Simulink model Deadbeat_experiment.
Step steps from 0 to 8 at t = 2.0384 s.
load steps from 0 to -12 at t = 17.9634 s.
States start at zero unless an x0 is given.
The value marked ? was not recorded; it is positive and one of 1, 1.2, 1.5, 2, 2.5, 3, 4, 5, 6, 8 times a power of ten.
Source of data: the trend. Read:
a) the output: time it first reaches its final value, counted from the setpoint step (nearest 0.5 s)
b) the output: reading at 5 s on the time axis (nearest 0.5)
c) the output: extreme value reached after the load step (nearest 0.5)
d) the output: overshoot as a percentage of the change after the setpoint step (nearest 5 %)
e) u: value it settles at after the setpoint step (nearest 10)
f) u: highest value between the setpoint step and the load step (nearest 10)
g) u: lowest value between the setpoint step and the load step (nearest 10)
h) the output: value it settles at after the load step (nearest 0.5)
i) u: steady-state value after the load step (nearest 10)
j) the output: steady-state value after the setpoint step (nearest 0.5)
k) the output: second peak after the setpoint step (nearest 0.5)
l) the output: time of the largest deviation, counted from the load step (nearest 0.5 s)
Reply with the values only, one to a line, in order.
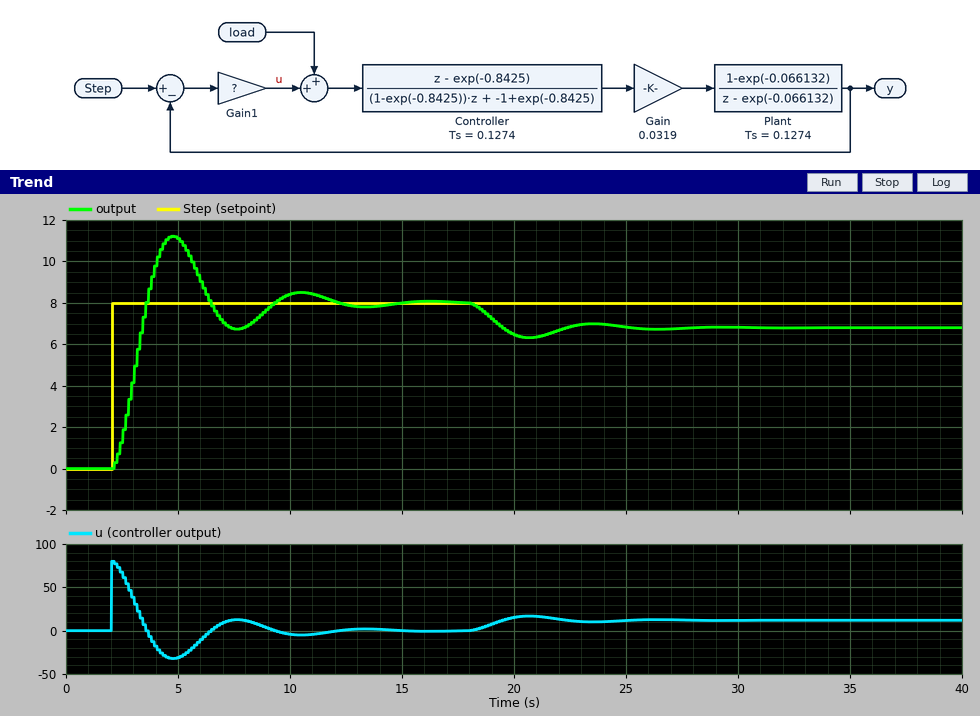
1.5 s
11.0
6.5
40 %
0
80
-30
7.0
10
8.0
8.5
2.5 s
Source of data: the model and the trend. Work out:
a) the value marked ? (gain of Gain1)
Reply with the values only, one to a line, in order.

10
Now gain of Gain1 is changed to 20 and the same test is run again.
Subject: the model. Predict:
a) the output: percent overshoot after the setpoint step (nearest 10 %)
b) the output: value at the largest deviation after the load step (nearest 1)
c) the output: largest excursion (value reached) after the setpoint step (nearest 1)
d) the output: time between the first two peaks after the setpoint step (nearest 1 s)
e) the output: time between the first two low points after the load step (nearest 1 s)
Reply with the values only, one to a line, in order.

50 %
7
12
4 s
4 s
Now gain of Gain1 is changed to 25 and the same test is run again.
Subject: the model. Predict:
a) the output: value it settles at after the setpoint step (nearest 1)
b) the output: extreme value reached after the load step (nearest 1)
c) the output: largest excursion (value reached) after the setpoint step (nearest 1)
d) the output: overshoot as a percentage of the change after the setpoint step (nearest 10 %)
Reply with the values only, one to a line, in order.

8
7
12
50 %
